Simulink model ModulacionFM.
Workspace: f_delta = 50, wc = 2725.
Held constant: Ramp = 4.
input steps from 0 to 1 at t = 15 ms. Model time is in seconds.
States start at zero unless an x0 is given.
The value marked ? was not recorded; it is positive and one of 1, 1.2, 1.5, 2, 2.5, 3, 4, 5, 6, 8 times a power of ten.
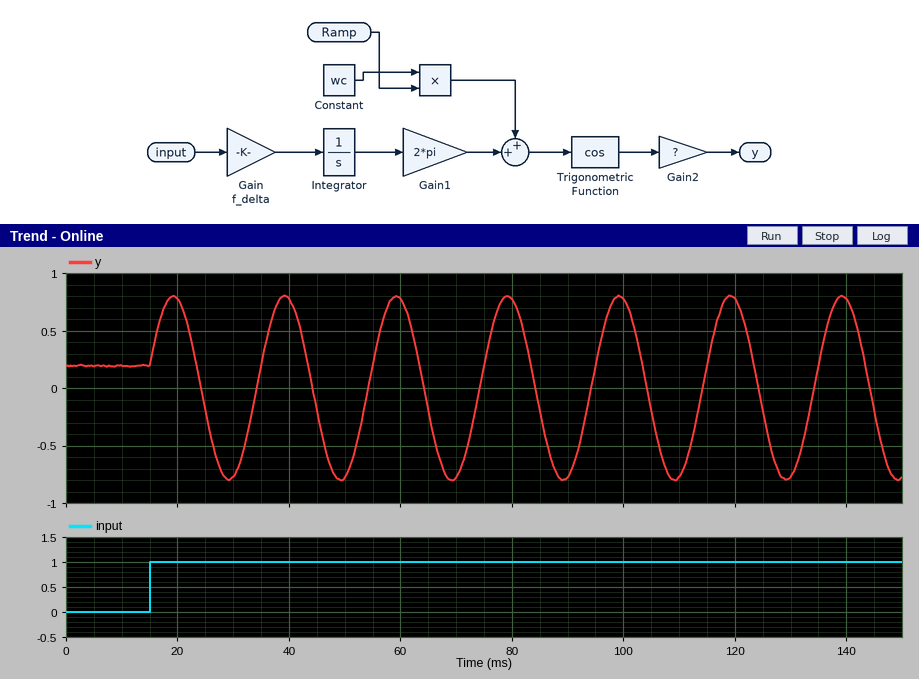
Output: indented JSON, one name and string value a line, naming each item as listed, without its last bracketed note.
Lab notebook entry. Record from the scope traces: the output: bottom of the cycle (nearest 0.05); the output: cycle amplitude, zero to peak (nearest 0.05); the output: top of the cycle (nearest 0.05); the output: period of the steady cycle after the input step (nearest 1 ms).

{
  "the output: bottom of the cycle": "-0.80",
  "the output: cycle amplitude, zero to peak": "0.80",
  "the output: top of the cycle": "0.80",
  "the output: period of the steady cycle after the input step": "20 ms"
}
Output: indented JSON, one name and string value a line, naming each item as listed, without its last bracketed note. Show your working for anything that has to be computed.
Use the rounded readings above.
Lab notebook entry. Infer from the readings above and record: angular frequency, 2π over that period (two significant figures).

{
  "angular frequency, 2π over that period": "2π / 20 = 0.31 rad/ms"
}
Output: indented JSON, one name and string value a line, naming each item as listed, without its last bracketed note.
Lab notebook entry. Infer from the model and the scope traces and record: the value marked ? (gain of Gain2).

{
  "the value marked ?": "0.8"
}
